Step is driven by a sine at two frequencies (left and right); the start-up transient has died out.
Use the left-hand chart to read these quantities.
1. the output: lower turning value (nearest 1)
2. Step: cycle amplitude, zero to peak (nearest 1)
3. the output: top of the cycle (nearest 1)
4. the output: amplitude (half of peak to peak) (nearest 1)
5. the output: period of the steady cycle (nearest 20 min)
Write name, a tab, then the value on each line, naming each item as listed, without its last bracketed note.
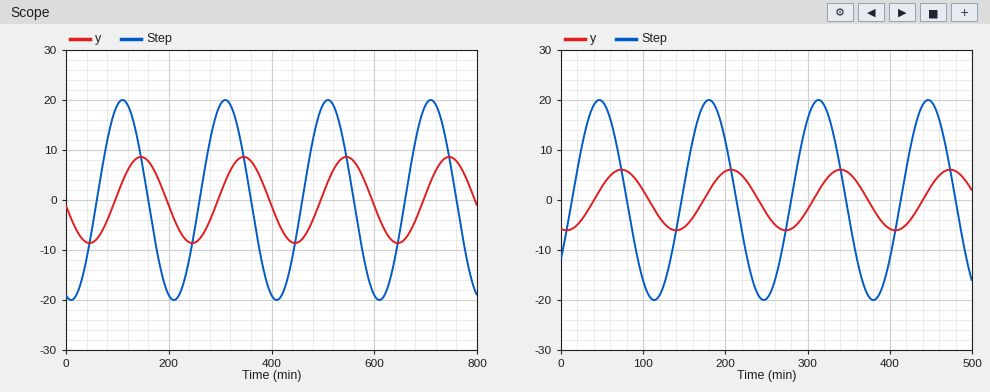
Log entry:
the output: lower turning value	-9
Step: cycle amplitude, zero to peak	20
the output: top of the cycle	9
the output: amplitude (half of peak to peak)	9
the output: period of the steady cycle	200 min
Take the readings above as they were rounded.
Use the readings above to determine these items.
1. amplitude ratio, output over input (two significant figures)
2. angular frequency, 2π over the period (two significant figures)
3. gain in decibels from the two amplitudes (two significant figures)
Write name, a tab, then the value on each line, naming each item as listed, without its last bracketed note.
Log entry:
amplitude ratio, output over input	0.45
angular frequency, 2π over the period	0.031 rad/min
gain in decibels from the two amplitudes	-6.9 dB
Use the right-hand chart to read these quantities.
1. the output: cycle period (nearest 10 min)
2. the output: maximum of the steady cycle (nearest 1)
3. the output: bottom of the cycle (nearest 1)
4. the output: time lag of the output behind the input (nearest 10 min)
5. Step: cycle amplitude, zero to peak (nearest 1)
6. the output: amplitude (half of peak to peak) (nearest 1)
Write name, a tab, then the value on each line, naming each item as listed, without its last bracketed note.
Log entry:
the output: cycle period	130 min
the output: maximum of the steady cycle	6
the output: bottom of the cycle	-6
the output: time lag of the output behind the input	30 min
Step: cycle amplitude, zero to peak	20
the output: amplitude (half of peak to peak)	6
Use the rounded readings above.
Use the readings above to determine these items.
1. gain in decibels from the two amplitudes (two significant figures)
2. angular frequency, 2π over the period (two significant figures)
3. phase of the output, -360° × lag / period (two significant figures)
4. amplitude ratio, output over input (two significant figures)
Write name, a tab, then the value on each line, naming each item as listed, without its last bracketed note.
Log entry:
gain in decibels from the two amplitudes	-10 dB
angular frequency, 2π over the period	0.048 rad/min
phase of the output, -360° × lag / period	-83°
amplitude ratio, output over input	0.30
